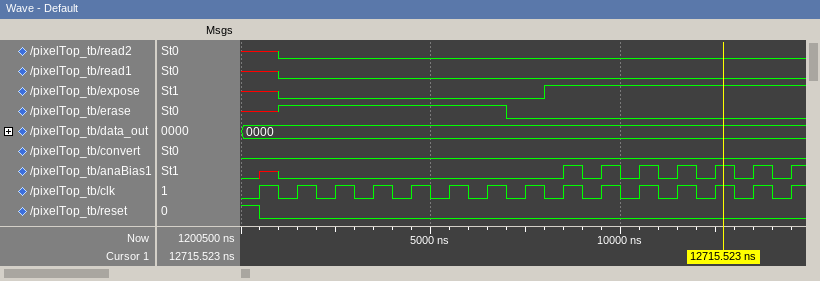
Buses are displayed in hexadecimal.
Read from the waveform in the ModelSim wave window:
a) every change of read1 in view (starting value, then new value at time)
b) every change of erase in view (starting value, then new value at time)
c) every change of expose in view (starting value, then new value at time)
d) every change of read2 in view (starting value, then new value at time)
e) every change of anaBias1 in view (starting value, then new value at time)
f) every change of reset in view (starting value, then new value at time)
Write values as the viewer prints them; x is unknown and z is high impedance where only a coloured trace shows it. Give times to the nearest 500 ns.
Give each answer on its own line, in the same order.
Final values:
x, 0 at 1000 ns
x, 1 at 1000 ns, 0 at 7000 ns
x, 0 at 1000 ns, 1 at 8000 ns
x, 0 at 1000 ns
0, x at 500 ns, 0 at 1000 ns, 1 at 8500 ns, 0 at 9000 ns, 1 at 9500 ns, 0 at 10000 ns, 1 at 10500 ns, 0 at 11000 ns, 1 at 11500 ns, 0 at 12000 ns, 1 at 12500 ns, 0 at 13000 ns, 1 at 13500 ns, 0 at 14000 ns, 1 at 14500 ns
1, 0 at 500 ns
